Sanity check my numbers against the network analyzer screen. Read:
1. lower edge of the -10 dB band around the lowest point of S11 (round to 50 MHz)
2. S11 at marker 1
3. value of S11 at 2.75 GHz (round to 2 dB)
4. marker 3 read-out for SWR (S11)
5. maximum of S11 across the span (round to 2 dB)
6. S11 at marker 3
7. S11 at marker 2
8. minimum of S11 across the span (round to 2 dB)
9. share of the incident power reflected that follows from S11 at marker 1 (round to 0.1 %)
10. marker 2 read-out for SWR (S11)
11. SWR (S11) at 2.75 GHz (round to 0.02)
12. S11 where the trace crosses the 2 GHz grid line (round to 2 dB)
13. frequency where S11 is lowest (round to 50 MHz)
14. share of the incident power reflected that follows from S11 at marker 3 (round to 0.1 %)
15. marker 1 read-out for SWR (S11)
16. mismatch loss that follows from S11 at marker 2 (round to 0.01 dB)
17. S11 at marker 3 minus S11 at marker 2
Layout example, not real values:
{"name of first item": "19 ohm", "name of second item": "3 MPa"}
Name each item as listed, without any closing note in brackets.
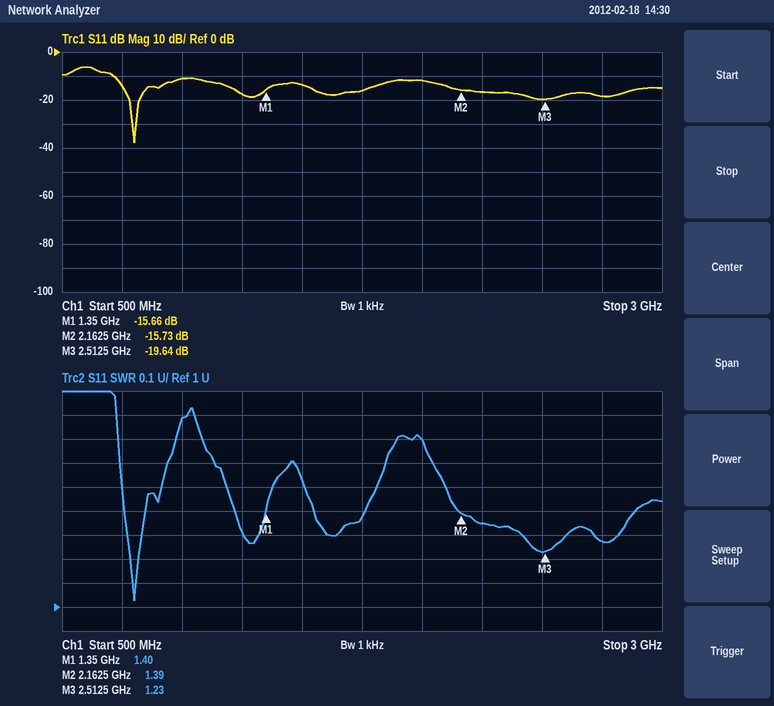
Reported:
{"lower edge of the -10 dB band around the lowest point of S11": "700 MHz", "S11 at marker 1": "-15.66 dB", "value of S11 at 2.75 GHz": "-18 dB", "marker 3 read-out for SWR": "1.23", "maximum of S11 across the span": "-6 dB", "S11 at marker 3": "-19.64 dB", "S11 at marker 2": "-15.73 dB", "minimum of S11 across the span": "-38 dB", "share of the incident power reflected that follows from S11 at marker 1": "2.7 %", "marker 2 read-out for SWR": "1.39", "SWR (S11) at 2.75 GHz": "1.28", "S11 where the trace crosses the 2 GHz grid line": "-12 dB", "frequency where S11 is lowest": "800 MHz", "share of the incident power reflected that follows from S11 at marker 3": "1.1 %", "marker 1 read-out for SWR": "1.40", "mismatch loss that follows from S11 at marker 2": "0.12 dB", "S11 at marker 3 minus S11 at marker 2": "-3.91 dB"}
